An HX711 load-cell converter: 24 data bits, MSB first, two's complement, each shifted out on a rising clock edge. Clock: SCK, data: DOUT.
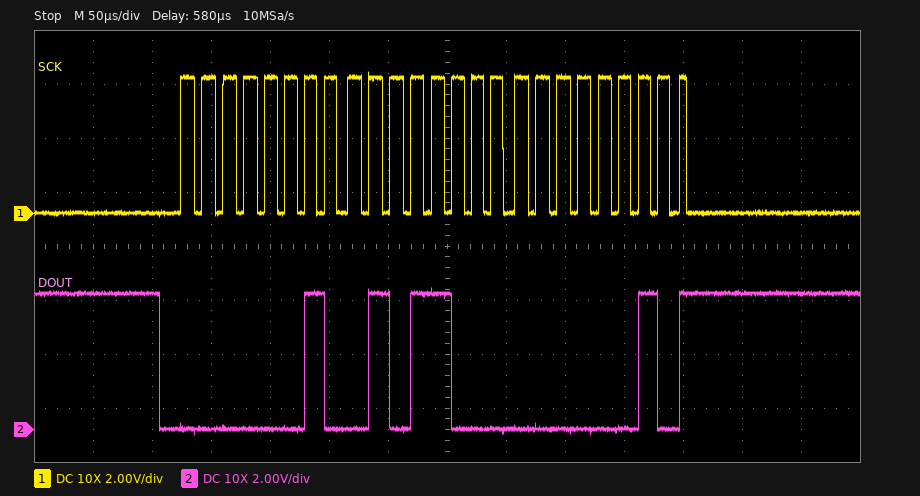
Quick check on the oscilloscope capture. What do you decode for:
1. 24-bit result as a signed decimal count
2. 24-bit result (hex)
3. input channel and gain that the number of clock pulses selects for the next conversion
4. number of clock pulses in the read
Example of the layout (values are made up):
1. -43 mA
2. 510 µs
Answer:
1. 153602
2. 0x025802
3. channel A, gain 128
4. 25
